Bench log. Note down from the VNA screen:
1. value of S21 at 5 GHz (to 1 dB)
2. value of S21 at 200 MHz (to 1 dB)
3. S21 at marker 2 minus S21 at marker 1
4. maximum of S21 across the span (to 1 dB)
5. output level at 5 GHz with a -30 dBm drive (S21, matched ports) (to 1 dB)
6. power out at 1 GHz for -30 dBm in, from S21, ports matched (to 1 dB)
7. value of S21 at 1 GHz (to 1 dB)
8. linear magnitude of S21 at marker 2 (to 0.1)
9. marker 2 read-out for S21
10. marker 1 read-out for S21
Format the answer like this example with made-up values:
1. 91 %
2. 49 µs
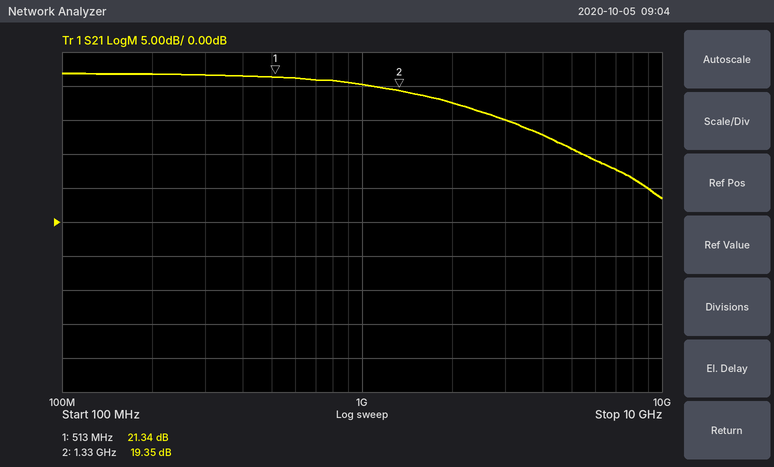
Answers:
1. 11 dB
2. 22 dB
3. -1.99 dB
4. 22 dB
5. -19 dBm
6. -10 dBm
7. 20 dB
8. 9.3
9. 19.35 dB
10. 21.34 dB
